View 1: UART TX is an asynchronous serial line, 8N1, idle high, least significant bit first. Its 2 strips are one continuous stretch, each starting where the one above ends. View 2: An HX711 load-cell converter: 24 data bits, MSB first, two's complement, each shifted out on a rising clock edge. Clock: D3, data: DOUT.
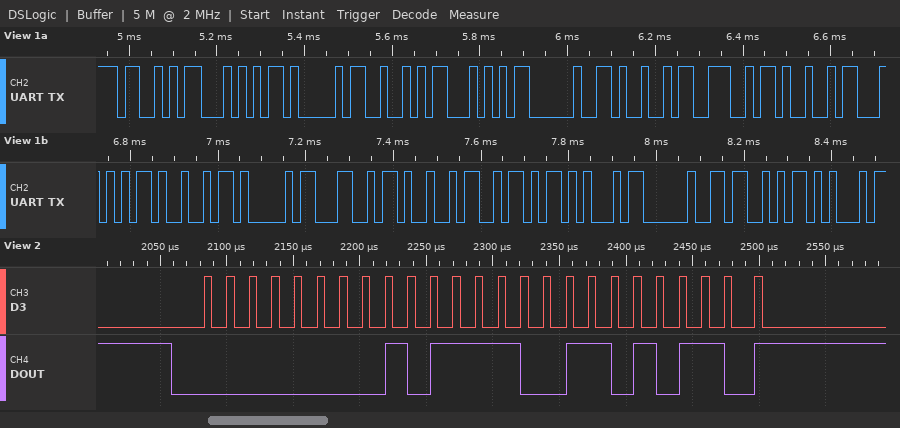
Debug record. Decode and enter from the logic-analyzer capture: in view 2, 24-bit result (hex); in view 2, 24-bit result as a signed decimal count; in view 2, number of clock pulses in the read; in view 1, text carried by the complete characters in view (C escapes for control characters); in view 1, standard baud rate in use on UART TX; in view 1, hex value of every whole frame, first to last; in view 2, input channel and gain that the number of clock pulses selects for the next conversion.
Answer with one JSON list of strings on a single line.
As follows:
["0x00BCD6", "48342", "25", "\"START INITIALIZE SE\"", "57600 baud", "53 54 41 52 54 20 49 4E 49 54 49 41 4C 49 5A 45 20 53 45", "channel A, gain 128"]
